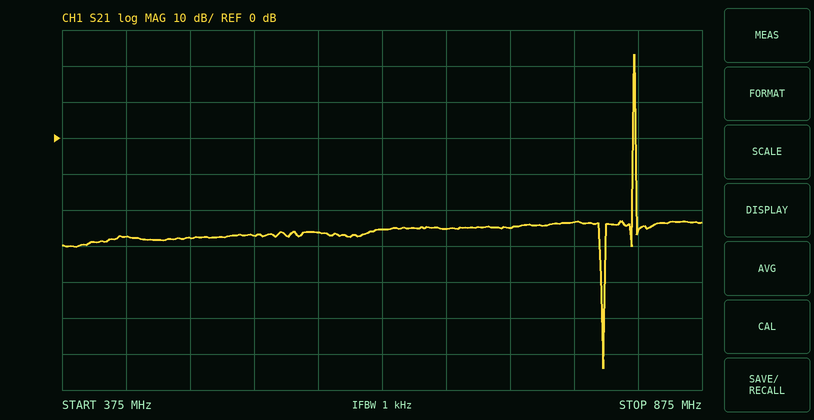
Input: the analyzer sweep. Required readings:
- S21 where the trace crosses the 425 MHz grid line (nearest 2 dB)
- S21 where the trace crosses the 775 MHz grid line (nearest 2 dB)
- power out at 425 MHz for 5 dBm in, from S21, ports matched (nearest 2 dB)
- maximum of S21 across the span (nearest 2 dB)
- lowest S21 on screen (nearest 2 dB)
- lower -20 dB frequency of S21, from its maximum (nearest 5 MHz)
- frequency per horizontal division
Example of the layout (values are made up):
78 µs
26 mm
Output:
-28 dB
-24 dB
-22 dBm
24 dB
-64 dB
820 MHz
50 MHz
